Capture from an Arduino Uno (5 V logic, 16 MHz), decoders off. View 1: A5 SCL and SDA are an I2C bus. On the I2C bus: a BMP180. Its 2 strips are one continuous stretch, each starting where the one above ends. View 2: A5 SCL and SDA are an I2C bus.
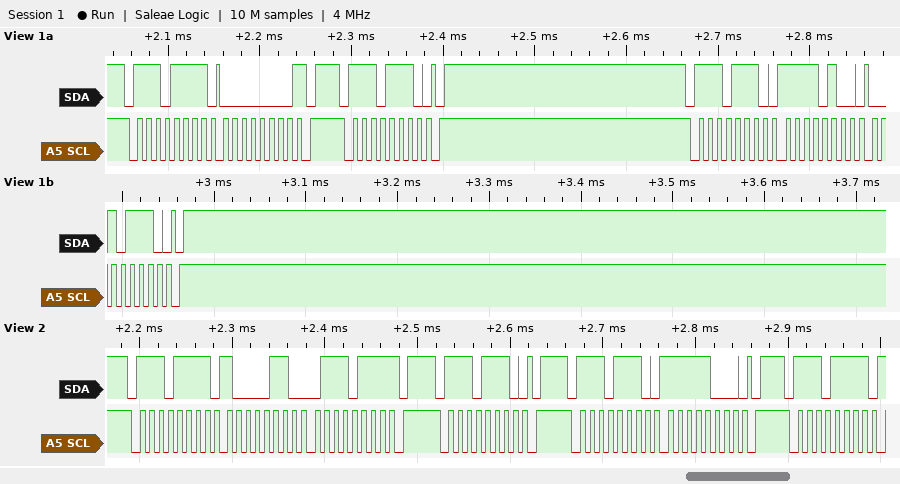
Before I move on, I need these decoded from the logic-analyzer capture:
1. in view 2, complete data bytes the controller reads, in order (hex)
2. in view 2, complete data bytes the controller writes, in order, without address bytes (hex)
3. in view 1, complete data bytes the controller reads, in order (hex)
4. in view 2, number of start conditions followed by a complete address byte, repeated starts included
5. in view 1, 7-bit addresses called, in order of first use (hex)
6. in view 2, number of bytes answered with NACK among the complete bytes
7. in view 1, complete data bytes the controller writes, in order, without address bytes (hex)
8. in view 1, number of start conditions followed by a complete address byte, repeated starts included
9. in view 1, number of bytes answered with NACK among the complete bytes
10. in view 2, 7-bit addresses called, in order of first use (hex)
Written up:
86 77
F8
00
4
0x77
1
F4 2E
3
1
0x77
